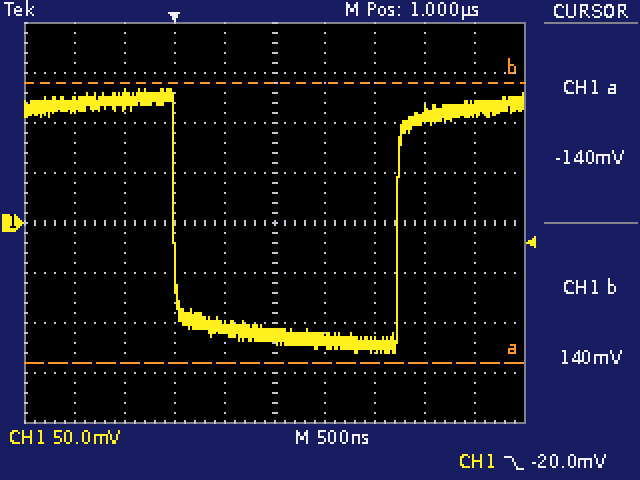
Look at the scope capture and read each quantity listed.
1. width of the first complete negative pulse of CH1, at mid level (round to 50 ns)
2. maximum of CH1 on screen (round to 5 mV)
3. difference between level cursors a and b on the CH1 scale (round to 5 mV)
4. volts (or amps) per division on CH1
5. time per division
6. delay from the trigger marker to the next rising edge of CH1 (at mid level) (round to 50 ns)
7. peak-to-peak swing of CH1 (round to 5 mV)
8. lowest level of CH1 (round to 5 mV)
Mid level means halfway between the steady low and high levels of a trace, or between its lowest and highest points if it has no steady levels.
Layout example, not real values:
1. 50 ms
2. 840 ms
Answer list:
1. 2.25 µs
2. 135 mV
3. 280 mV
4. 50 mV
5. 500 ns
6. 2.25 µs
7. 265 mV
8. -130 mV
